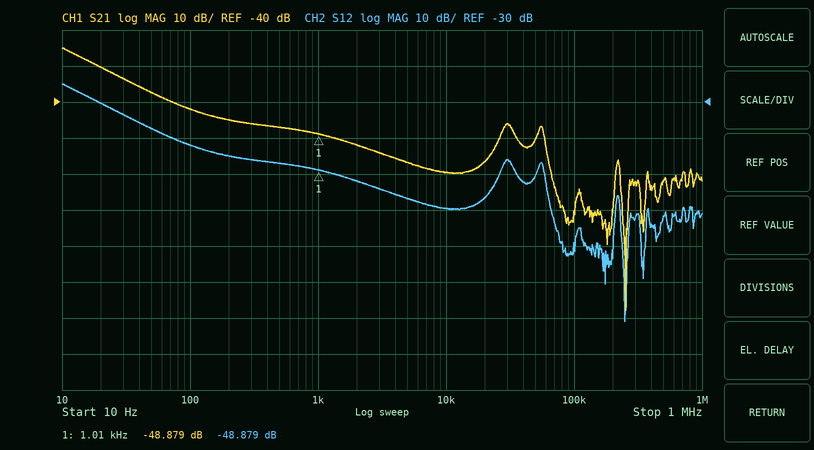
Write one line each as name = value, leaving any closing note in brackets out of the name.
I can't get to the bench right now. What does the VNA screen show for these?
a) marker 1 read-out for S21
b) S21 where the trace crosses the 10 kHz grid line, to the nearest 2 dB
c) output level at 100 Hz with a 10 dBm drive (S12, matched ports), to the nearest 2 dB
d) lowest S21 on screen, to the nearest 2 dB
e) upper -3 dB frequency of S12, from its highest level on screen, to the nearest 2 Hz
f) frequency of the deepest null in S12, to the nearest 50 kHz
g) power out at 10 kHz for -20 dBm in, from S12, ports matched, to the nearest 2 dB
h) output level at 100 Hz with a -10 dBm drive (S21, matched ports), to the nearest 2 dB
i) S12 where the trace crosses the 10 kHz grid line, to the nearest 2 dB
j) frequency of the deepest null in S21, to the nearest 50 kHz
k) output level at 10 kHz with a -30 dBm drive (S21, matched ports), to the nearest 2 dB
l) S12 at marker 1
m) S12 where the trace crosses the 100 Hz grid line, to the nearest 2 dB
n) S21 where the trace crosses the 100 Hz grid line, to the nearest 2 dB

marker 1 read-out for S21 = -48.879 dB
S21 where the trace crosses the 10 kHz grid line, to the nearest 2 dB = -60 dB
output level at 100 Hz with a 10 dBm drive (S12, matched ports), to the nearest 2 dB = -32 dBm
lowest S21 on screen, to the nearest 2 dB = -98 dB
upper -3 dB frequency of S12, from its highest level on screen, to the nearest 2 Hz = 14 Hz
frequency of the deepest null in S12, to the nearest 50 kHz = 250 kHz
power out at 10 kHz for -20 dBm in, from S12, ports matched, to the nearest 2 dB = -80 dBm
output level at 100 Hz with a -10 dBm drive (S21, matched ports), to the nearest 2 dB = -52 dBm
S12 where the trace crosses the 10 kHz grid line, to the nearest 2 dB = -60 dB
frequency of the deepest null in S21, to the nearest 50 kHz = 250 kHz
output level at 10 kHz with a -30 dBm drive (S21, matched ports), to the nearest 2 dB = -90 dBm
S12 at marker 1 = -48.879 dB
S12 where the trace crosses the 100 Hz grid line, to the nearest 2 dB = -42 dB
S21 where the trace crosses the 100 Hz grid line, to the nearest 2 dB = -42 dB
